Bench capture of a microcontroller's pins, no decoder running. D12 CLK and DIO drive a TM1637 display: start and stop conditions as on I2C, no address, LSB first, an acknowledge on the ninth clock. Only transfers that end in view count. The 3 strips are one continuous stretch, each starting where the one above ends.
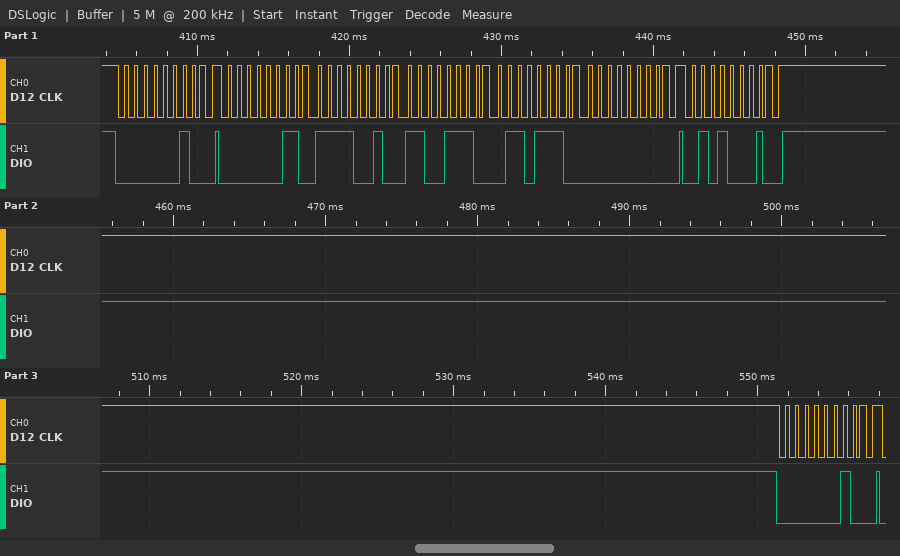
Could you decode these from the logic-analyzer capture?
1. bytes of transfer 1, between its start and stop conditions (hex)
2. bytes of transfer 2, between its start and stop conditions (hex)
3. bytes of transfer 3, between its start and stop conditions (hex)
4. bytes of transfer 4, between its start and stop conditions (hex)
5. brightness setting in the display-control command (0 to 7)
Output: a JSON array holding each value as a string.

["40", "C0 4F 73 76 00", "8A", "40", "2"]
